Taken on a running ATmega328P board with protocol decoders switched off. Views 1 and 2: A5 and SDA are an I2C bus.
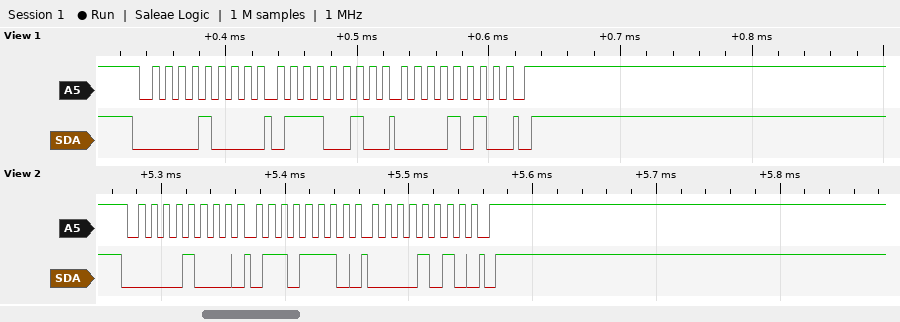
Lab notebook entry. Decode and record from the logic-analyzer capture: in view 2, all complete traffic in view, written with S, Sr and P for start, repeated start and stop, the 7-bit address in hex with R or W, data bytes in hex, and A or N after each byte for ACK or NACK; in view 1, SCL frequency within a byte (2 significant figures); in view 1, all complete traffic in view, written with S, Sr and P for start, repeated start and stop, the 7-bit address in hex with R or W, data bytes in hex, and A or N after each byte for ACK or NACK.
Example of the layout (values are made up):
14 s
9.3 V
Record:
S 04W A 6E A 0A A P
100 kHz
S 04W A 72 A 0A A P
